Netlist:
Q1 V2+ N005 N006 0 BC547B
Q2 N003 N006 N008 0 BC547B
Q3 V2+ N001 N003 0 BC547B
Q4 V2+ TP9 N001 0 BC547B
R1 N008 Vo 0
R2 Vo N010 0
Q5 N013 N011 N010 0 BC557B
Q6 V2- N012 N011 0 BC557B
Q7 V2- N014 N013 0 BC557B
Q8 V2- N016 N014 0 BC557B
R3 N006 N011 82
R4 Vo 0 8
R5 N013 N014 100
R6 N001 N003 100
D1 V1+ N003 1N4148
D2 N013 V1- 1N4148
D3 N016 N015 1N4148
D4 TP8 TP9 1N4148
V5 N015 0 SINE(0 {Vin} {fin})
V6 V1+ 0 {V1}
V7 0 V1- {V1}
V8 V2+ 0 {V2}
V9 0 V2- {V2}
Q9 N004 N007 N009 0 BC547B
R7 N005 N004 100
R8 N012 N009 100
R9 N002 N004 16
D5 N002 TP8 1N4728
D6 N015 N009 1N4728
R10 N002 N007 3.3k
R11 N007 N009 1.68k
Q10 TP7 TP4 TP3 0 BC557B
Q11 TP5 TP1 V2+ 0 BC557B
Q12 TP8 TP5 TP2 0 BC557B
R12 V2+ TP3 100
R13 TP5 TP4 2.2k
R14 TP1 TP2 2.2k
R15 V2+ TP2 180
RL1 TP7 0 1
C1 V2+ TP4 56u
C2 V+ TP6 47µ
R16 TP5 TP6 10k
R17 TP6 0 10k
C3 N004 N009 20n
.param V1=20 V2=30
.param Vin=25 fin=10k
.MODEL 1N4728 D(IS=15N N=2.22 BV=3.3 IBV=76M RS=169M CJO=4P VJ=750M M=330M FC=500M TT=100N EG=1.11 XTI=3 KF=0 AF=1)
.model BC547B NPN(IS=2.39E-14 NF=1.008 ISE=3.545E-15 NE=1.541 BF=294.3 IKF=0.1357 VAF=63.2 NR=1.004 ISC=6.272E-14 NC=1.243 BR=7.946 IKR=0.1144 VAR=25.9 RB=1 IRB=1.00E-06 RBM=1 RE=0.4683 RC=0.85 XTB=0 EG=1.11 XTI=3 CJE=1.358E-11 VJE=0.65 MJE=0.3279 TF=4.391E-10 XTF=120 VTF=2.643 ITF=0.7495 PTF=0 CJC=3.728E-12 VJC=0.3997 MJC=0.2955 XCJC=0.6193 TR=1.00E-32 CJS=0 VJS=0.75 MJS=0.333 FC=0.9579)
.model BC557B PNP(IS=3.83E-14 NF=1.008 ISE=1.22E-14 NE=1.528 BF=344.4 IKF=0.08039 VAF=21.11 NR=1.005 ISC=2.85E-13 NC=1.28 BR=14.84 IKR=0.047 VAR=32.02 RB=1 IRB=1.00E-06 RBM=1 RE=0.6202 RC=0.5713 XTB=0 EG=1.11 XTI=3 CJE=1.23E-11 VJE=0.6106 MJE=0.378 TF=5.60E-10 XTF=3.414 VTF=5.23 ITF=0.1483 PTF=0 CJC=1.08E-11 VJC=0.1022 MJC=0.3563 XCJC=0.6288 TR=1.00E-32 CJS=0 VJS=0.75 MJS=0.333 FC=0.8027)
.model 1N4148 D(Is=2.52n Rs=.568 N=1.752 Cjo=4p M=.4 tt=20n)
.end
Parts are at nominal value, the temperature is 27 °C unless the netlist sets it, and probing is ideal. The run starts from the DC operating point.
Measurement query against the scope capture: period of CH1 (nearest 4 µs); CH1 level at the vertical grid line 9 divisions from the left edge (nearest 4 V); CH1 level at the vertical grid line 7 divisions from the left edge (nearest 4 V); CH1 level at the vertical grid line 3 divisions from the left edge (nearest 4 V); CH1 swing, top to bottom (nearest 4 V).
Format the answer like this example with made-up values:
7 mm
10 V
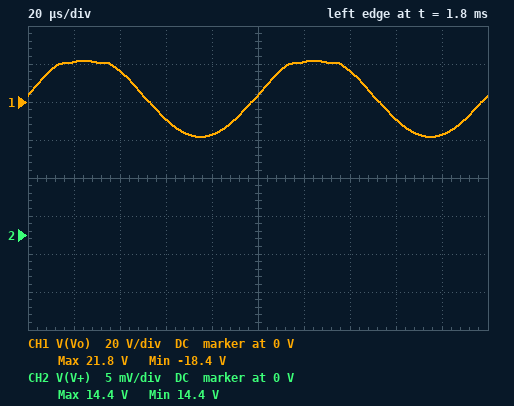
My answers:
100 µs
-16 V
16 V
-8 V
40 V
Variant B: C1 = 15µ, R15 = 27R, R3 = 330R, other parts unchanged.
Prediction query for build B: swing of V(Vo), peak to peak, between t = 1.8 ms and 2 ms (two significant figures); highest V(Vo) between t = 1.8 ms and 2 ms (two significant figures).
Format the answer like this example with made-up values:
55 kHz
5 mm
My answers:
41 V
23 V
